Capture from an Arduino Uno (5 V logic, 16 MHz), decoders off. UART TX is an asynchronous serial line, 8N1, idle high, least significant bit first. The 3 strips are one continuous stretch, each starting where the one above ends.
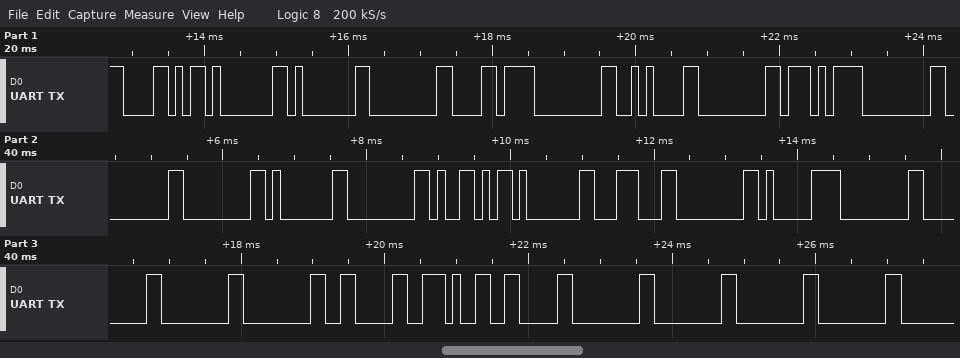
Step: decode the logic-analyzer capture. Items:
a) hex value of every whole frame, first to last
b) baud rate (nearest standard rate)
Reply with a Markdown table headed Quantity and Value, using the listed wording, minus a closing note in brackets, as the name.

| Quantity | Value |
|---|---|
| hex value of every whole frame, first to last | 58 01 01 00 D8 00 0A 00 D7 00 00 00 01 00 59 01 1C 00 C1 00 00 00 00 06 2E 06 00 00 00 00 |
| baud rate | 9600 baud |
